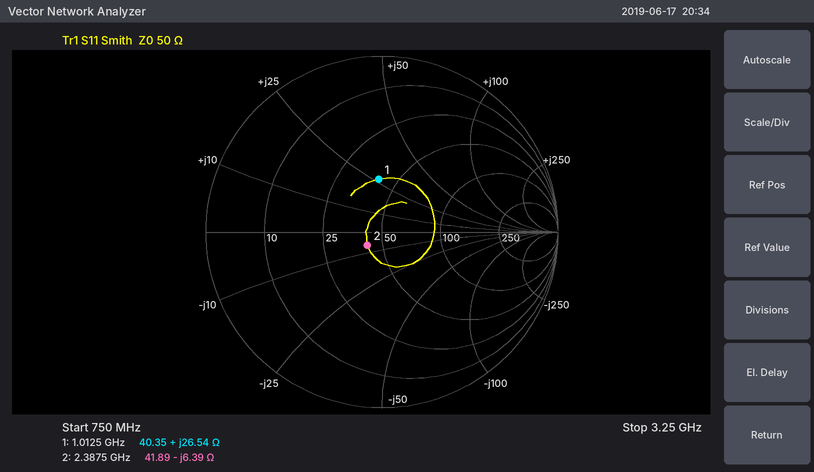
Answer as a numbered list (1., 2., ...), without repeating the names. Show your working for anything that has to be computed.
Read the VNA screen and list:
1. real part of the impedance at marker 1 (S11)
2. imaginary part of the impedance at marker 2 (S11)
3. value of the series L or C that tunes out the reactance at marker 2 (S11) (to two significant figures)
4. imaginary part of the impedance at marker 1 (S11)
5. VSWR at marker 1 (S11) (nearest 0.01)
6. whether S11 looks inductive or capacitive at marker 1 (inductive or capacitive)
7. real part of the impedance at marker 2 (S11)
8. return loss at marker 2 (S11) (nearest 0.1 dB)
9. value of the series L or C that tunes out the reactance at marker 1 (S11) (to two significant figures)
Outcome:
1. 40.35 Ω
2. -6.39 Ω
3. L = 6.39 Ω/(2π × 2.3875 GHz) ≈ 426 pH, so 430 pH to two significant figures
4. +26.54 Ω
5. 1.86
6. inductive
7. 41.89 Ω
8. 19.0 dB
9. C = 1/(2π × 1.0125 GHz × 26.54 Ω) ≈ 5.9 pF
